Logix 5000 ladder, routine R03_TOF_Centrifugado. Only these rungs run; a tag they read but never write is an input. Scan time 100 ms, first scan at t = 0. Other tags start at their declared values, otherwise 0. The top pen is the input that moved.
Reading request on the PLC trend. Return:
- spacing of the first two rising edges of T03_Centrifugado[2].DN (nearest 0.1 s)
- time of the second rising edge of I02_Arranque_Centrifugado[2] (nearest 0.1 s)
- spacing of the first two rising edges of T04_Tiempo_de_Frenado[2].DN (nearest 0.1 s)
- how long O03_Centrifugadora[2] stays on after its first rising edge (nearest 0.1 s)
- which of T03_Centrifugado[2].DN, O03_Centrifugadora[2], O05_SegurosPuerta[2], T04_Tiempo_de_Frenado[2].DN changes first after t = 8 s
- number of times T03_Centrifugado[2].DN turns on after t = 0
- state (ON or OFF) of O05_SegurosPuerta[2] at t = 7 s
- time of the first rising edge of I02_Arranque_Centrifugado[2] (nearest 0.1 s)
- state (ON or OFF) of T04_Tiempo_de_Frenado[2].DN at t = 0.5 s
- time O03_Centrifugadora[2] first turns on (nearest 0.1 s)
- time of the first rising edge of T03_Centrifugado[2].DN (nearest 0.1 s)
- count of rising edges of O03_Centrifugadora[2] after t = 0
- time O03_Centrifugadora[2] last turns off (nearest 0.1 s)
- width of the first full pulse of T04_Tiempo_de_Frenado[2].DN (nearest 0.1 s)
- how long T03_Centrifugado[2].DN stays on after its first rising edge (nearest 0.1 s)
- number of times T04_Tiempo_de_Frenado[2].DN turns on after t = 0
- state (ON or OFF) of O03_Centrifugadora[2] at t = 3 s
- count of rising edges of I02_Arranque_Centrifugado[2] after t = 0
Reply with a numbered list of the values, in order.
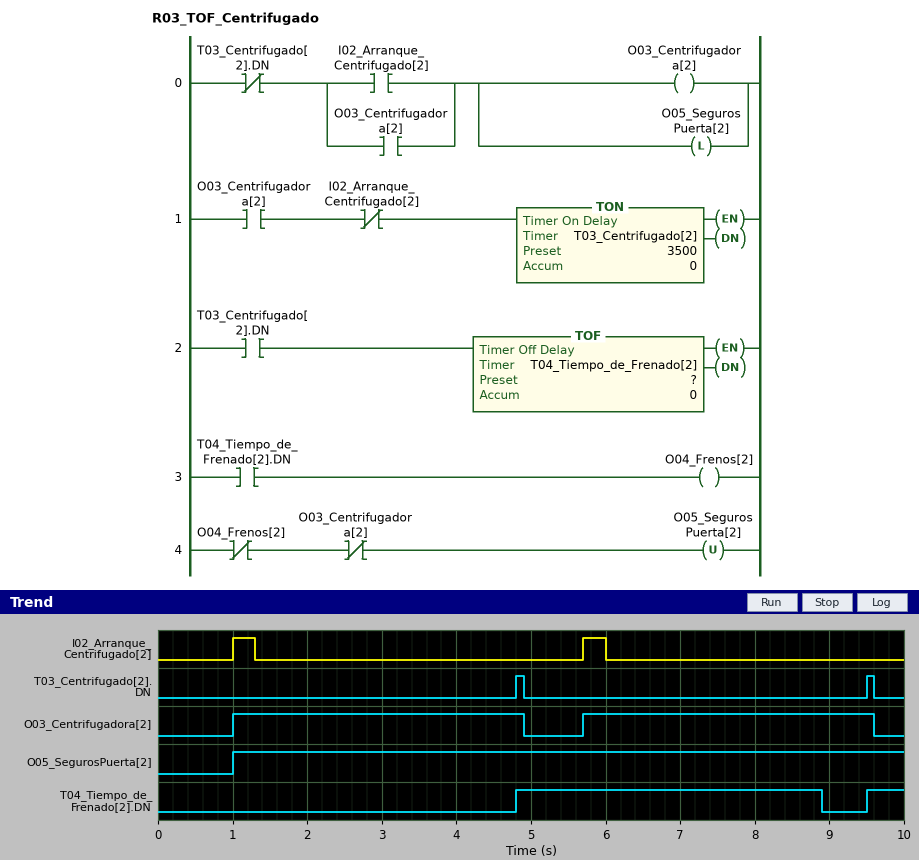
1. 4.7 s
2. 5.7 s
3. 4.7 s
4. 3.9 s
5. T04_Tiempo_de_Frenado[2].DN
6. 2
7. ON
8. 1.0 s
9. OFF
10. 1.0 s
11. 4.8 s
12. 2
13. 9.6 s
14. 4.1 s
15. 0.1 s
16. 2
17. ON
18. 2
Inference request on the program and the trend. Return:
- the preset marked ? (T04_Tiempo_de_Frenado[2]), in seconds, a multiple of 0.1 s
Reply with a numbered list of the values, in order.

1. 4.0 s
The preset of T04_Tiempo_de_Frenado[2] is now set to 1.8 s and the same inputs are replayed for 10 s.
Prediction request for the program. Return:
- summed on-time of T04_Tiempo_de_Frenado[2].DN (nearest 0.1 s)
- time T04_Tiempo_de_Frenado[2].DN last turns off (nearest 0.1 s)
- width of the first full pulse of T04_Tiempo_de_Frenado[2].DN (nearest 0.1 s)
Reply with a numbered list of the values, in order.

1. 2.4 s
2. 6.7 s
3. 1.9 s
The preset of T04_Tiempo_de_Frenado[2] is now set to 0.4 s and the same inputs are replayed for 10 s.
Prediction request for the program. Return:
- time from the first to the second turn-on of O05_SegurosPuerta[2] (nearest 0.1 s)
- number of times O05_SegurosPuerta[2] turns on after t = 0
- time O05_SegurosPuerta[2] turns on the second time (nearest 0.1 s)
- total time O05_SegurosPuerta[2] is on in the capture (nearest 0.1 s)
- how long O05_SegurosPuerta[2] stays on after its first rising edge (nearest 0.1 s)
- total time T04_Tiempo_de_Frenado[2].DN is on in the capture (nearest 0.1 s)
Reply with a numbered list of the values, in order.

1. 4.7 s
2. 2
3. 5.7 s
4. 8.6 s
5. 4.3 s
6. 1.0 s
